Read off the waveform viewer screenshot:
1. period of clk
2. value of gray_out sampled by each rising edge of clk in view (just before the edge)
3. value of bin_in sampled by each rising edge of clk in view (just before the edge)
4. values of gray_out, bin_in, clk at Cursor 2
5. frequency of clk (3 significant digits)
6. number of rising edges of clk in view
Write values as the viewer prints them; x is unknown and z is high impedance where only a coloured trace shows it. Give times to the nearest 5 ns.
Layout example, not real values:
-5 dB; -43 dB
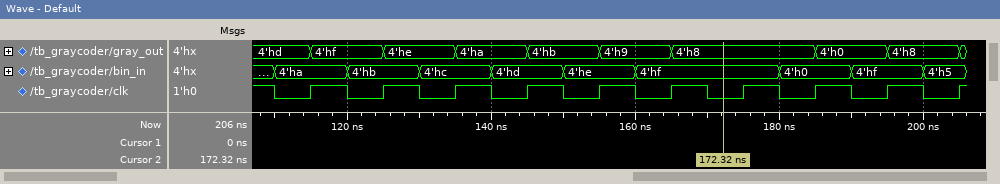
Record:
10 ns; 4'hd, 4'hf, 4'he, 4'ha, 4'hb, 4'h9, 4'h8, 4'h8, 4'h0, 4'h8; 4'ha, 4'hb, 4'hc, 4'hd, 4'he, 4'hf, 4'hf, 4'h0, 4'hf, 4'h5; gray_out=4'h8, bin_in=4'hf, clk=0; 100 MHz; 10
